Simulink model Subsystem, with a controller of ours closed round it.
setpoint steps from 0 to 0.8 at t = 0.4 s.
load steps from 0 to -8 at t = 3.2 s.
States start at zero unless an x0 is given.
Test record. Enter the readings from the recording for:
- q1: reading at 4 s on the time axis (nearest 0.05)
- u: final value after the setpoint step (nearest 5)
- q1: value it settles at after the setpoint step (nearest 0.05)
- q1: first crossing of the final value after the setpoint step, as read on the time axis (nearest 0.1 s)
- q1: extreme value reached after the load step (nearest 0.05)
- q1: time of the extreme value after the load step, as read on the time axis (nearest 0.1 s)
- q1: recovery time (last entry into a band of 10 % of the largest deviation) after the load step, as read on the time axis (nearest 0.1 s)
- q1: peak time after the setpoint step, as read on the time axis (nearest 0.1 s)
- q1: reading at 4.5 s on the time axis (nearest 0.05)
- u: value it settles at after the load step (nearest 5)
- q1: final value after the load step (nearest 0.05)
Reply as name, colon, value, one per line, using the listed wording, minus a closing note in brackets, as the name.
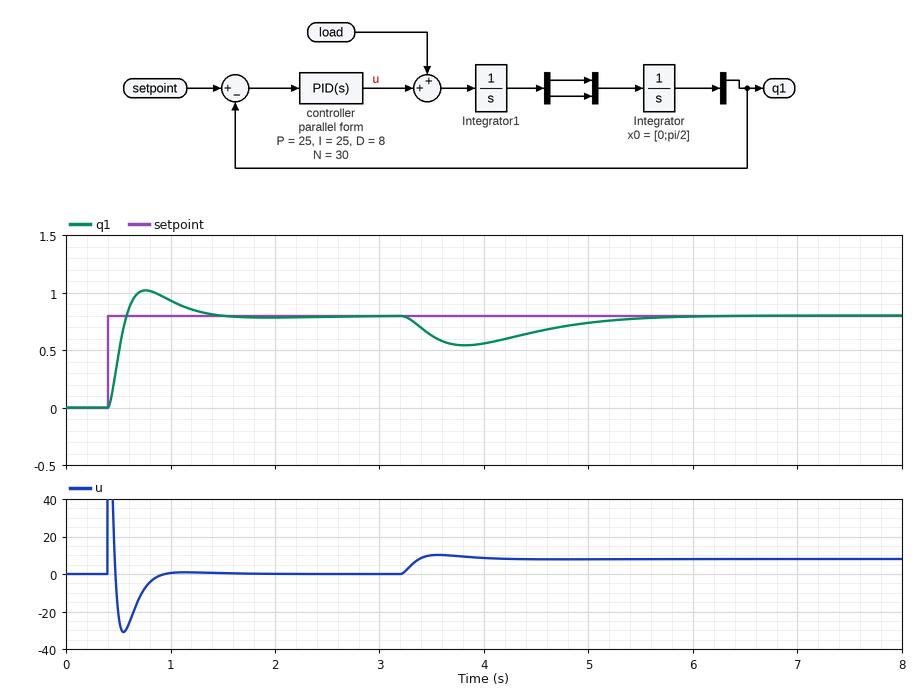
q1: reading at 4 s on the time axis: 0.55
u: final value after the setpoint step: 0
q1: value it settles at after the setpoint step: 0.80
q1: first crossing of the final value after the setpoint step, as read on the time axis: 0.6 s
q1: extreme value reached after the load step: 0.55
q1: time of the extreme value after the load step, as read on the time axis: 3.8 s
q1: recovery time (last entry into a band of 10 % of the largest deviation) after the load step, as read on the time axis: 5.5 s
q1: peak time after the setpoint step, as read on the time axis: 0.8 s
q1: reading at 4.5 s on the time axis: 0.65
u: value it settles at after the load step: 10
q1: final value after the load step: 0.80
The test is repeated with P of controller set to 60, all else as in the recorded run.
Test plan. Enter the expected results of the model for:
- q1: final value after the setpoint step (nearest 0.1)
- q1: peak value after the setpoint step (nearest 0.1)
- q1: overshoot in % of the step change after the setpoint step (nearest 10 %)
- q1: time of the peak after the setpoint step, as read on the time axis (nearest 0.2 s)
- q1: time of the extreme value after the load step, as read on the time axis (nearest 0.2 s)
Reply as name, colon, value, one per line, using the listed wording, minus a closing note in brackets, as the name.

q1: final value after the setpoint step: 0.8
q1: peak value after the setpoint step: 1.1
q1: overshoot in % of the step change after the setpoint step: 40 %
q1: time of the peak after the setpoint step, as read on the time axis: 0.6 s
q1: time of the extreme value after the load step, as read on the time axis: 3.6 s
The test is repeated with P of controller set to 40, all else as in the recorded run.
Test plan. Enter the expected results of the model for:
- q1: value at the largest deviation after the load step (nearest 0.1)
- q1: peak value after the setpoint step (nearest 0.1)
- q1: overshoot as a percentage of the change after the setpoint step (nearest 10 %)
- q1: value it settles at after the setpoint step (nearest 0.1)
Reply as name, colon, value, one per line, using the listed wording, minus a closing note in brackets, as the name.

q1: value at the largest deviation after the load step: 0.6
q1: peak value after the setpoint step: 1.1
q1: overshoot as a percentage of the change after the setpoint step: 30 %
q1: value it settles at after the setpoint step: 0.8
